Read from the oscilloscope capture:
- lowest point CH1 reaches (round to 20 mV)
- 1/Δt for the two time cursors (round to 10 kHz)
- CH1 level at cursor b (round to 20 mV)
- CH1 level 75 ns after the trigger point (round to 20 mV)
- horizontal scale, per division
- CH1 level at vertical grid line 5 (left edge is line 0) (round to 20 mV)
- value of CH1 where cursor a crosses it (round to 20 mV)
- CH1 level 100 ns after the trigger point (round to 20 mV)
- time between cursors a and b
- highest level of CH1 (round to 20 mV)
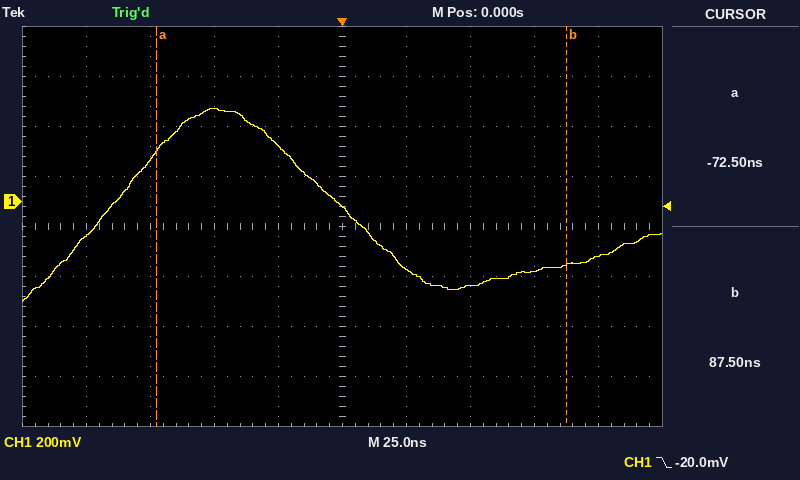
-400 mV
6.25 MHz
-260 mV
-280 mV
25 ns
-20 mV
200 mV
-220 mV
160.0 ns
380 mV
